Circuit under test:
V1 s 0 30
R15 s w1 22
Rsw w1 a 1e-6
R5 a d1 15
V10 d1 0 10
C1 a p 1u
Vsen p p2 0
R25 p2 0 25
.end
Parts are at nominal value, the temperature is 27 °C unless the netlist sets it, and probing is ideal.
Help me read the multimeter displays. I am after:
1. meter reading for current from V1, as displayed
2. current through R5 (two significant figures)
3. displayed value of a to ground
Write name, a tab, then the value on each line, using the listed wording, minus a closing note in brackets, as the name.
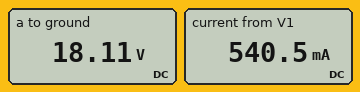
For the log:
meter reading for current from V1, as displayed	540.5 mA
current through R5	540 mA
displayed value of a to ground	18.11 V
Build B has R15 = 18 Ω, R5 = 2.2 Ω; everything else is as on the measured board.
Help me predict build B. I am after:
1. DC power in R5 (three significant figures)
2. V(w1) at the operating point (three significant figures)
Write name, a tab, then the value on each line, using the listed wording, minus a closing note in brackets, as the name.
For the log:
DC power in R5	2.16 W
V(w1) at the operating point	12.2 V
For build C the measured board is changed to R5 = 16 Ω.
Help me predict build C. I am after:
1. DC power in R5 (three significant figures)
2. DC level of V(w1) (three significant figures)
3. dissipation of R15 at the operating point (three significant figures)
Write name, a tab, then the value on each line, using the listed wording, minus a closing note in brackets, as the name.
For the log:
DC power in R5	4.43 W
DC level of V(w1)	18.4 V
dissipation of R15 at the operating point	6.09 W
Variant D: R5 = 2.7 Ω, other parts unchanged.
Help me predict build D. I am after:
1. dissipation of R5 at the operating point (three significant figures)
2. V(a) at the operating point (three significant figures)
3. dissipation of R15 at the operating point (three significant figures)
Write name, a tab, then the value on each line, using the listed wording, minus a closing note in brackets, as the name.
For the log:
dissipation of R5 at the operating point	1.77 W
V(a) at the operating point	12.2 V
dissipation of R15 at the operating point	14.4 W
